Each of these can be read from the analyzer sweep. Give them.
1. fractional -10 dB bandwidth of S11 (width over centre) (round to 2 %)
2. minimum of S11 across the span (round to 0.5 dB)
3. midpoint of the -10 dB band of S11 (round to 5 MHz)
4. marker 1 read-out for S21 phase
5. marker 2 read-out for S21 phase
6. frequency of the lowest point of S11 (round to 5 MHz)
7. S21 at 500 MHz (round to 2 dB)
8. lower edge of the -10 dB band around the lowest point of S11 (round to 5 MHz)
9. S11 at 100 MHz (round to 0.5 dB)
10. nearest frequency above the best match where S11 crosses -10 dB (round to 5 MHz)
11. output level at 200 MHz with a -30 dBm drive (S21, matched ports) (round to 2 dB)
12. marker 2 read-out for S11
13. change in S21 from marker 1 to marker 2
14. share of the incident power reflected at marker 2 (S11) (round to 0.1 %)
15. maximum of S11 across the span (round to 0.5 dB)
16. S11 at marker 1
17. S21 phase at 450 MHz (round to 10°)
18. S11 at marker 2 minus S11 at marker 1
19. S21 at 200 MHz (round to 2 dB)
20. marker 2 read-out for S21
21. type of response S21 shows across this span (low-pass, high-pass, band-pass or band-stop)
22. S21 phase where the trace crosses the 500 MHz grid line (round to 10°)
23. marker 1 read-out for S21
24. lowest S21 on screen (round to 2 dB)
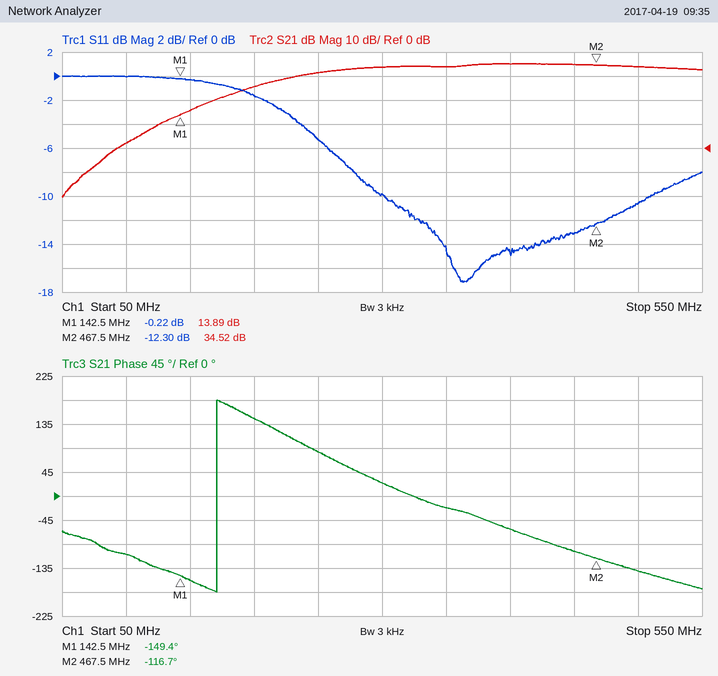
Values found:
52 %
-17.0 dB
405 MHz
-149.4°
-116.7°
365 MHz
34 dB
300 MHz
0.0 dB
510 MHz
-4 dBm
-12.30 dB
20.63 dB
5.9 %
0.0 dB
-0.22 dB
-100°
-12.08 dB
26 dB
34.52 dB
high-pass
-140°
13.89 dB
-20 dB
